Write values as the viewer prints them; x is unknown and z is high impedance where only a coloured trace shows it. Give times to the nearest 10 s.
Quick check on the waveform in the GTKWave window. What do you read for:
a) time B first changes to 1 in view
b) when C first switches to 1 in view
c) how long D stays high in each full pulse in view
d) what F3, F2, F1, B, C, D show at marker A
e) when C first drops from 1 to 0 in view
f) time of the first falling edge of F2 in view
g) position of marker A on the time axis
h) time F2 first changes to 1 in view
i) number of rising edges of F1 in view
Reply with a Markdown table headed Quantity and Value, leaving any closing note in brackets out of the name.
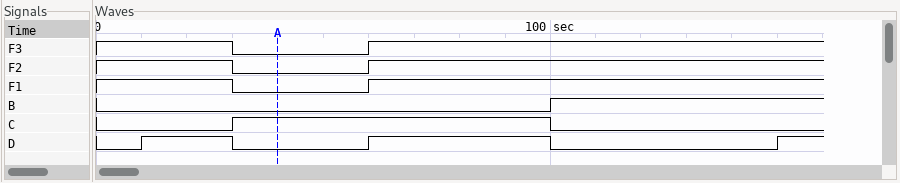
| Quantity | Value |
|---|---|
| time B first changes to 1 in view | 100 s |
| when C first switches to 1 in view | 30 s |
| how long D stays high in each full pulse in view | 20 s, 40 s |
| what F3, F2, F1, B, C, D show at marker A | F3=0, F2=0, F1=0, B=0, C=1, D=0 |
| when C first drops from 1 to 0 in view | 100 s |
| time of the first falling edge of F2 in view | 30 s |
| position of marker A on the time axis | 40 s |
| time F2 first changes to 1 in view | 60 s |
| number of rising edges of F1 in view | 1 |
